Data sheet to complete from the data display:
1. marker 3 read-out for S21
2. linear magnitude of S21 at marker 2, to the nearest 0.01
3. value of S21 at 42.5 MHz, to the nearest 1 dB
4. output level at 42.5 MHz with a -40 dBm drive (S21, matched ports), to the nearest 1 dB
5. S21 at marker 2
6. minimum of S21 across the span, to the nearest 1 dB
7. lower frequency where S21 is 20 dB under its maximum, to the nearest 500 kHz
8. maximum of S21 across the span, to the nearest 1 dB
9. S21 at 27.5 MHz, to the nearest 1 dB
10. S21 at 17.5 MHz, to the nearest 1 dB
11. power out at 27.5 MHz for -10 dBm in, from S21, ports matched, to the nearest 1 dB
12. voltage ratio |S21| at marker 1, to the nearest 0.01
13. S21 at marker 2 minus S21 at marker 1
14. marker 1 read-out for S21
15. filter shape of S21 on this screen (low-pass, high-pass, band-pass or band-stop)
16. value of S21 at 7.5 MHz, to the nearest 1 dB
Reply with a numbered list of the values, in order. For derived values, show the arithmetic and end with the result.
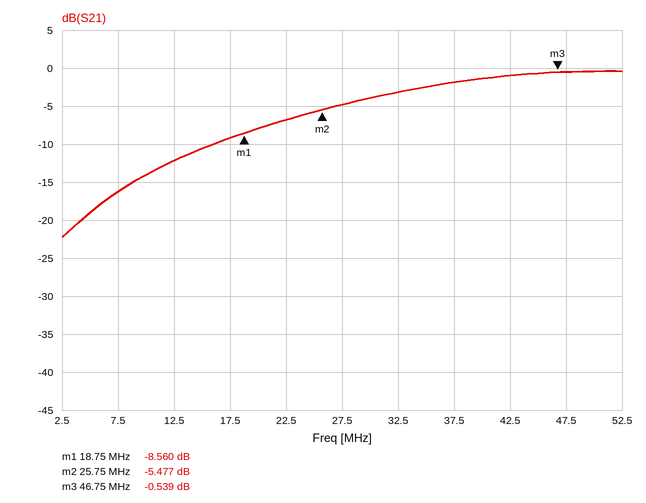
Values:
1. -0.539 dB
2. 10^(-5.477/20) ≈ 0.53
3. -1 dB
4. -40 dBm + (-1 dB) = -41 dBm
5. -5.477 dB
6. -22 dB
7. 4.0 MHz
8. 0 dB
9. -5 dB
10. -9 dB
11. -10 dBm + (-5 dB) = -15 dBm
12. 10^(-8.56/20) ≈ 0.37
13. -5.477 − (-8.56) = 3.083 dB
14. -8.560 dB
15. high-pass
16. -16 dB
